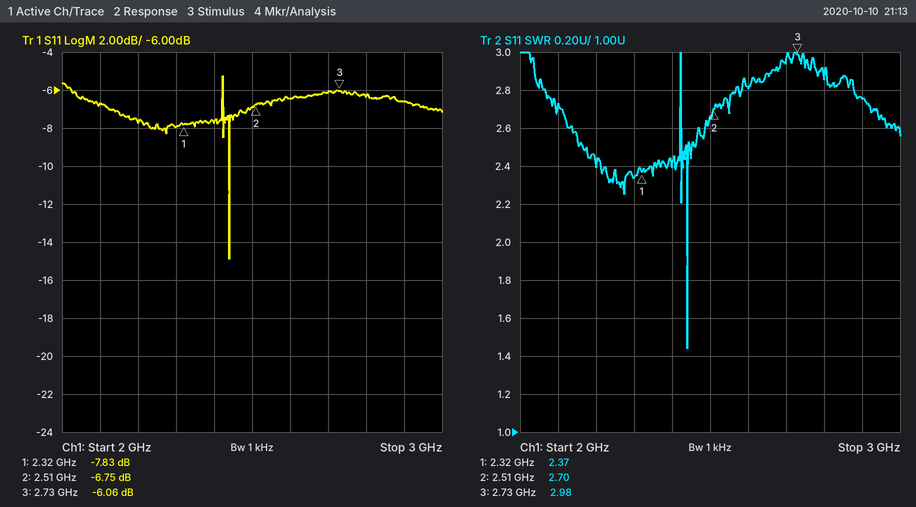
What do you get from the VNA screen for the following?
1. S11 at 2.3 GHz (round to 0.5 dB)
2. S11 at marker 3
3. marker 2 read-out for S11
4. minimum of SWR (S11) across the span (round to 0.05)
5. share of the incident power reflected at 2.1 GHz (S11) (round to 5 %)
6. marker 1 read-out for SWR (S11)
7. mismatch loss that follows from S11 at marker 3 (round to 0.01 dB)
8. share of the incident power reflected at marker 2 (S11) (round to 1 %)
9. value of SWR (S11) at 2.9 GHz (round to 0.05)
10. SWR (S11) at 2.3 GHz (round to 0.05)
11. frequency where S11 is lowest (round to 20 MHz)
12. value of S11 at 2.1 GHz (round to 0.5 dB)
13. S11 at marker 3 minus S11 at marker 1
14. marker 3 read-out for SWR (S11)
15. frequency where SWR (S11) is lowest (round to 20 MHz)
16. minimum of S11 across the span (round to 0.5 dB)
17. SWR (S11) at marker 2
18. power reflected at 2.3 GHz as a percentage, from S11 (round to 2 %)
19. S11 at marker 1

-8.0 dB
-6.06 dB
-6.75 dB
1.45
20 %
2.37
1.24 dB
21 %
2.75
2.35
2.44 GHz
-6.5 dB
1.77 dB
2.98
2.44 GHz
-15.0 dB
2.70
16 %
-7.83 dB
